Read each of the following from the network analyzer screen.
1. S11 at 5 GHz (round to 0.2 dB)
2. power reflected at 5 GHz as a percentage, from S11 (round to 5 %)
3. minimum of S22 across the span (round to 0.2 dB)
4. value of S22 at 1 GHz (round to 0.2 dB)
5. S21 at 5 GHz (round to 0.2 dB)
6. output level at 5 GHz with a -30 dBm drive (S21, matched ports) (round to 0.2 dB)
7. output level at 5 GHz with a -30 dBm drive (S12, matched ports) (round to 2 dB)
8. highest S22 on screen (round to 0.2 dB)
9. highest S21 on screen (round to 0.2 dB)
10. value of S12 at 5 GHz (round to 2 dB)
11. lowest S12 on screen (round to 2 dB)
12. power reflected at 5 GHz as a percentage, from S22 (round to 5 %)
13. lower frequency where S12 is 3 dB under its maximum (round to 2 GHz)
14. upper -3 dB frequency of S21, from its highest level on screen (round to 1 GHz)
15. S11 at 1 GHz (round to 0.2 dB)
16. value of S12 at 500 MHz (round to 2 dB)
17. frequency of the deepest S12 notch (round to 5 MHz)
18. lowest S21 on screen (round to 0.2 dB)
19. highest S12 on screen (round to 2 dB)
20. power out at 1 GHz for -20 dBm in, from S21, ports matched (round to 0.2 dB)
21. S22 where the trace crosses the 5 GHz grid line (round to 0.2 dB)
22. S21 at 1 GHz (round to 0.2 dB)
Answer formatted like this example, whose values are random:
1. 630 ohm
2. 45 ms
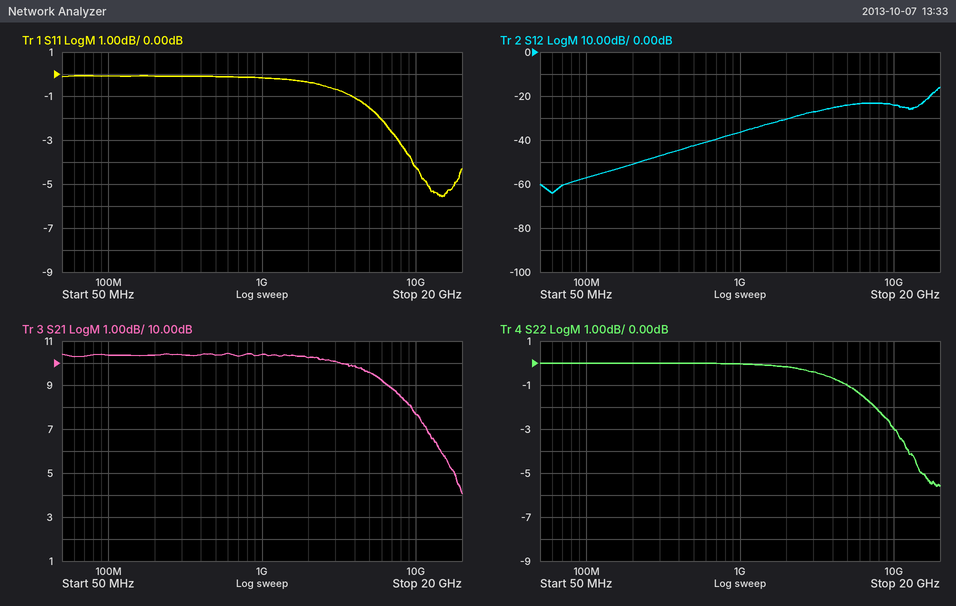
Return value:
1. -1.6 dB
2. 70 %
3. -5.6 dB
4. 0.0 dB
5. 9.6 dB
6. -20.4 dBm
7. -54 dBm
8. 0.0 dB
9. 10.4 dB
10. -24 dB
11. -64 dB
12. 80 %
13. 18 GHz
14. 11 GHz
15. -0.2 dB
16. -42 dB
17. 60 MHz
18. 4.0 dB
19. -16 dB
20. -9.6 dBm
21. -1.0 dB
22. 10.4 dB
